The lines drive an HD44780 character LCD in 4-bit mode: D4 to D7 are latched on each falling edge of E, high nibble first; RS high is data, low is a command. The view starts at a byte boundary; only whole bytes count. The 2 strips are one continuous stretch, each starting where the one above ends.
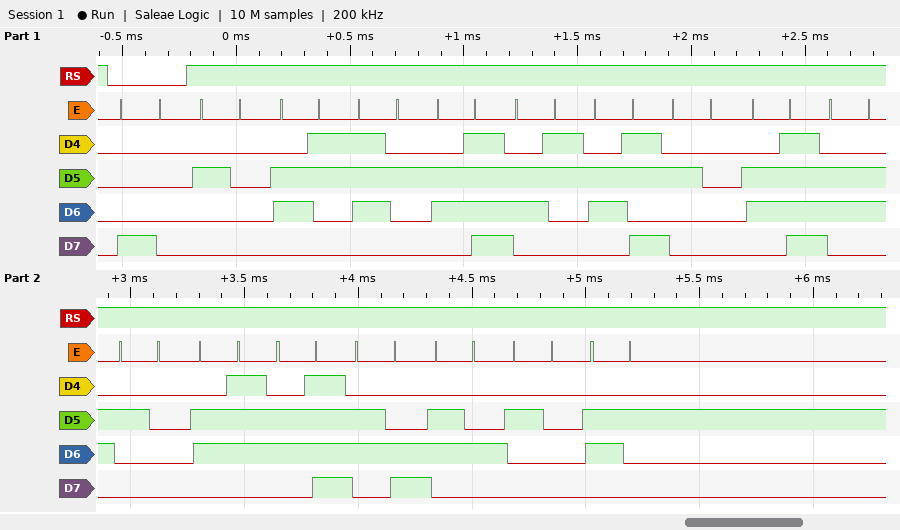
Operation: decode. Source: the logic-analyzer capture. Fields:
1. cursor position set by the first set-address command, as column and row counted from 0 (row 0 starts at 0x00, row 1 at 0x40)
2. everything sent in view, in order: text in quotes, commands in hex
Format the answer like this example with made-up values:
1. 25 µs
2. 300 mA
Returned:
1. column 0, row 0
2. 0x80 " crock of gold b"
